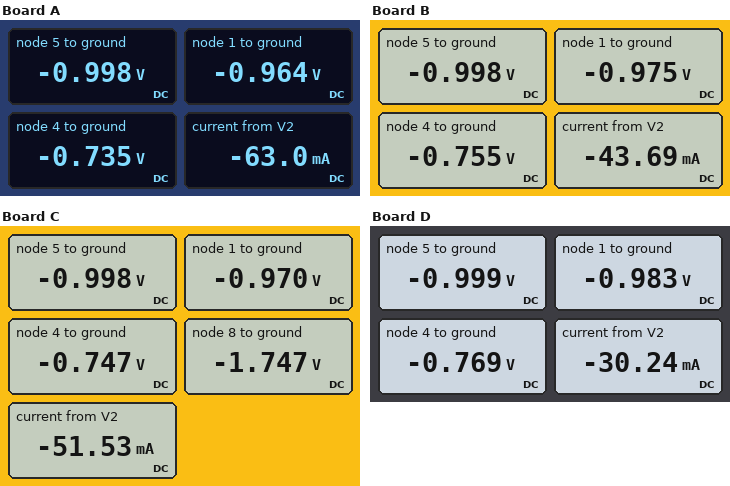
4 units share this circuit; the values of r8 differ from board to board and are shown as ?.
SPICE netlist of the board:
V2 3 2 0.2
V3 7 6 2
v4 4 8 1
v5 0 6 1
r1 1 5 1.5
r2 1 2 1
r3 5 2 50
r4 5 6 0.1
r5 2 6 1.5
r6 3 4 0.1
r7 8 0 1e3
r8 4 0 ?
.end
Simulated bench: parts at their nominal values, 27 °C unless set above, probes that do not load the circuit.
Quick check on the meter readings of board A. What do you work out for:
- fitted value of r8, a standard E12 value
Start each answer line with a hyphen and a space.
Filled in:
- 12 Ω
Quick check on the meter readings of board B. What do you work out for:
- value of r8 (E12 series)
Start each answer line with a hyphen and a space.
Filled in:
- 18 Ω
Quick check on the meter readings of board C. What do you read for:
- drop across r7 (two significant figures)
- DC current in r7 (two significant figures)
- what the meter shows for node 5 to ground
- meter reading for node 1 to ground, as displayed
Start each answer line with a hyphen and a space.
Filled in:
- 1.7 V
- 1.7 mA
- -0.998 V
- -0.970 V
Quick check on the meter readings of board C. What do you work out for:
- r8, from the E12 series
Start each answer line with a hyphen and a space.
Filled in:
- 15 Ω
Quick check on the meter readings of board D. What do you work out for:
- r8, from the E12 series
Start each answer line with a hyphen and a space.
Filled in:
- 27 Ω
